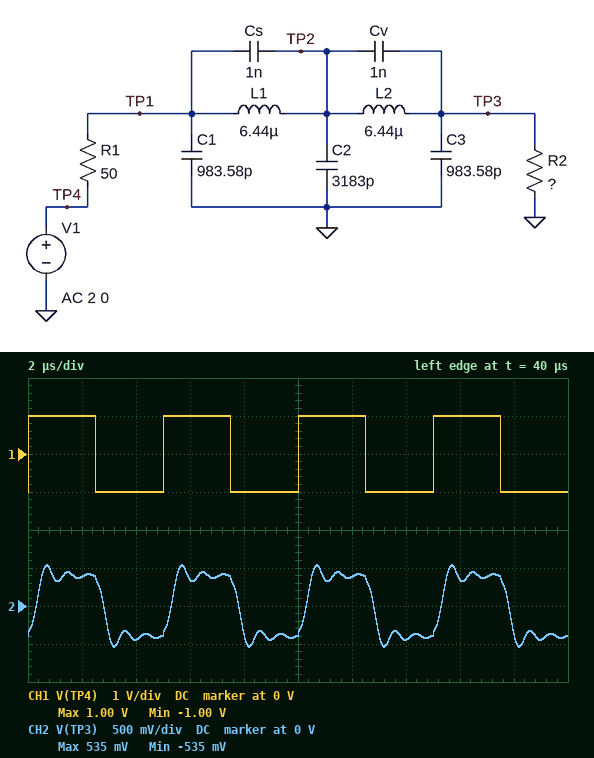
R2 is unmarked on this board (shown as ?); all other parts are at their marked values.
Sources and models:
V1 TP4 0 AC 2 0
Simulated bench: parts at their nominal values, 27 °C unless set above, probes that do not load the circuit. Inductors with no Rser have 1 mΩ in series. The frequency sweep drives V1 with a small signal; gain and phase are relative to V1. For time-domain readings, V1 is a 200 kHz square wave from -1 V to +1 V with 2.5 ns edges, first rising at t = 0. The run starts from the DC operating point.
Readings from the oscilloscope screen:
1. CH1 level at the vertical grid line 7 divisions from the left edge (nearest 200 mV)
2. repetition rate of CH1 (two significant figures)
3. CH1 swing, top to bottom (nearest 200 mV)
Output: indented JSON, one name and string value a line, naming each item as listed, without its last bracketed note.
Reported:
{
  "CH1 level at the vertical grid line 7 divisions from the left edge": "-1.0 V",
  "repetition rate of CH1": "200 kHz",
  "CH1 swing, top to bottom": "2.0 V"
}
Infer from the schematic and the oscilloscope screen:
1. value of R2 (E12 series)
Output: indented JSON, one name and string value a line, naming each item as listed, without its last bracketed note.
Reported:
{
  "value of R2": "33 Ω"
}
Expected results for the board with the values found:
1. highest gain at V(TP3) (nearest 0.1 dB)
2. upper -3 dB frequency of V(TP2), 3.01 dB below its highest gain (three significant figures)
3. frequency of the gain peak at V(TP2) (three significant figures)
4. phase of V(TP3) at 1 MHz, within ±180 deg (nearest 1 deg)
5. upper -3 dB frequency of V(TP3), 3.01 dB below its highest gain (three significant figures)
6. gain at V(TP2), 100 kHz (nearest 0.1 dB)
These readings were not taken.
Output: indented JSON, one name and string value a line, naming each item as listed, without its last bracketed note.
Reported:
{
  "highest gain at V(TP3)": "-8.0 dB",
  "upper -3 dB frequency of V(TP2), 3.01 dB below its highest gain": "1.41 MHz",
  "frequency of the gain peak at V(TP2)": "1.27 MHz",
  "phase of V(TP3) at 1 MHz, within ±180 deg": "-113 deg",
  "upper -3 dB frequency of V(TP3), 3.01 dB below its highest gain": "1.35 MHz",
  "gain at V(TP2), 100 kHz": "-8.0 dB"
}
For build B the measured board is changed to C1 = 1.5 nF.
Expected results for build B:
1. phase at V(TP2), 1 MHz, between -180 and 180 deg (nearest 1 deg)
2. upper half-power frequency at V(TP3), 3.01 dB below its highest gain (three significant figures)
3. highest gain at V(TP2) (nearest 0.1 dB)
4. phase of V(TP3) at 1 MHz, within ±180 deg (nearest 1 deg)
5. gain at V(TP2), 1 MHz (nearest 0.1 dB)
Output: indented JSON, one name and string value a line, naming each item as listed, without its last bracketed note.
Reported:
{
  "phase at V(TP2), 1 MHz, between -180 and 180 deg": "-50 deg",
  "upper half-power frequency at V(TP3), 3.01 dB below its highest gain": "1.36 MHz",
  "highest gain at V(TP2)": "0.2 dB",
  "phase of V(TP3) at 1 MHz, within ±180 deg": "-118 deg",
  "gain at V(TP2), 1 MHz": "-3.3 dB"
}
